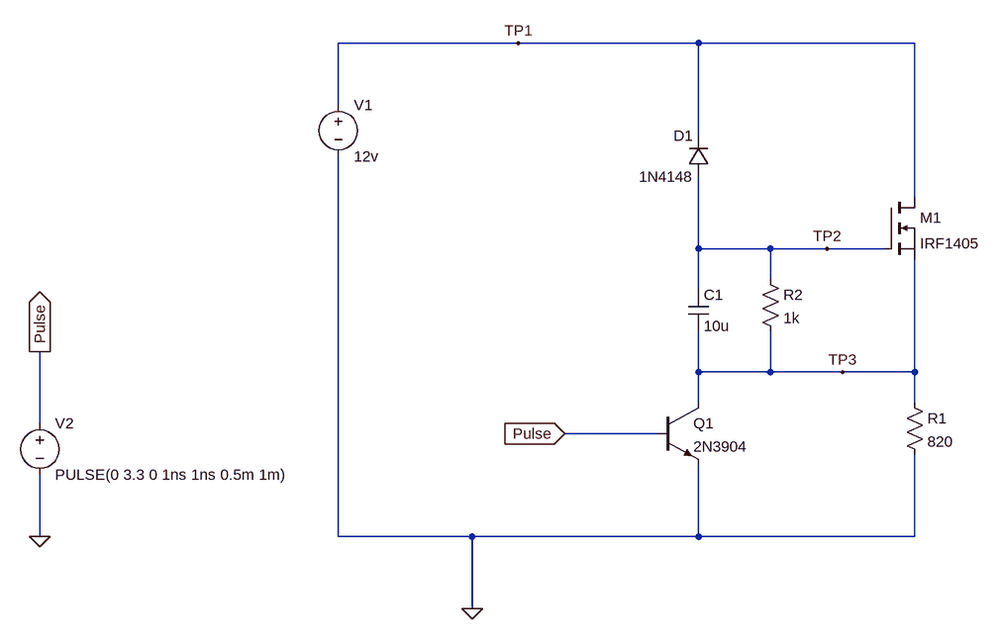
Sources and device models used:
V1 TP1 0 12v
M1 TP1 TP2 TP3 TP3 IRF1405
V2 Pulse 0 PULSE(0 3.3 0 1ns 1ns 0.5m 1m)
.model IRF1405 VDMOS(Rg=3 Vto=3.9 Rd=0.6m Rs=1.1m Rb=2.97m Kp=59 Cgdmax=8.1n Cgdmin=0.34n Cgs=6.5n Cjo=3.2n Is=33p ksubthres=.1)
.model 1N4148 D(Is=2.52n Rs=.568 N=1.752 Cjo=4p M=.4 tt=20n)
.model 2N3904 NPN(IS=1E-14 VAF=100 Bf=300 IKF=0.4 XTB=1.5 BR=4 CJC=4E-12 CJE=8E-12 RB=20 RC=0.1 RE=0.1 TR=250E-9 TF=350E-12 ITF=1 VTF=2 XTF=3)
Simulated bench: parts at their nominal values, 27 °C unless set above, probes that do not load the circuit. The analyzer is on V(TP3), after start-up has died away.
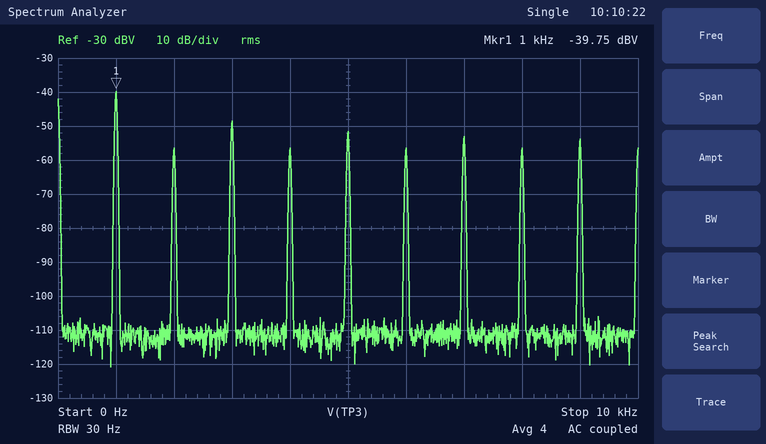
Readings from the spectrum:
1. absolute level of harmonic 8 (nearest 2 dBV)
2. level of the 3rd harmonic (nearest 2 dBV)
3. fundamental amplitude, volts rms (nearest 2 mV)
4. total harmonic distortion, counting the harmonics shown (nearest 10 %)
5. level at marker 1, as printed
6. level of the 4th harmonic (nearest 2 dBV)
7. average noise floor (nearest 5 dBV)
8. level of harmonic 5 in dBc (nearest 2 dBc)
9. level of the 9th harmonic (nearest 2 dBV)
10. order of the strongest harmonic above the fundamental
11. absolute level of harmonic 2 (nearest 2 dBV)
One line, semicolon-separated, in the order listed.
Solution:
-56 dBV; -48 dBV; 10 mV; 60 %; -39.75 dBV; -56 dBV; -110 dBV; -12 dBc; -54 dBV; 3; -56 dBV
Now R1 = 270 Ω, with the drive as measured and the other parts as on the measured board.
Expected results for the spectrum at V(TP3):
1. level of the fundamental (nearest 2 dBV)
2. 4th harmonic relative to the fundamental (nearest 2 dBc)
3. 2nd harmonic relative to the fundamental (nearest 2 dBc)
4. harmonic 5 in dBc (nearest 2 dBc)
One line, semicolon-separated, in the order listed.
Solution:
-40 dBV; -24 dBc; -24 dBc; -14 dBc
